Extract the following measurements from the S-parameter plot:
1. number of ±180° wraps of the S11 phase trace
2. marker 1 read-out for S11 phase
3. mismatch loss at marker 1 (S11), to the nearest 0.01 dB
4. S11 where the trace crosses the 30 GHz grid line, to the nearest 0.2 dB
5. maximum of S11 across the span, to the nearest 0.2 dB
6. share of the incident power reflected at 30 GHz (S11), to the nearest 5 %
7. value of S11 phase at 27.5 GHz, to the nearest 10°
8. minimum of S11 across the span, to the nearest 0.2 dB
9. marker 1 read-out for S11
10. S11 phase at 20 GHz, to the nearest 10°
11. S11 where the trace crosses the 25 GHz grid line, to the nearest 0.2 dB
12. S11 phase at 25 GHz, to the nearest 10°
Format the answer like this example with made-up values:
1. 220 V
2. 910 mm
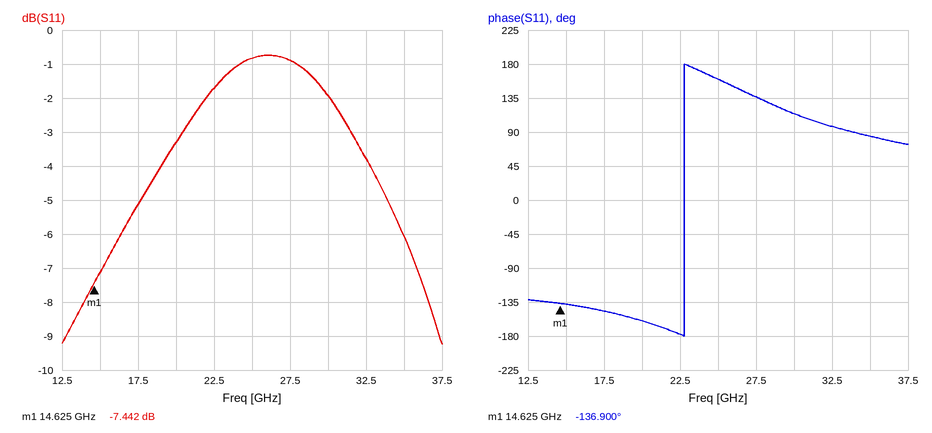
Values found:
1. 1
2. -136.900°
3. 0.86 dB
4. -2.0 dB
5. -0.8 dB
6. 65 %
7. 140°
8. -9.2 dB
9. -7.442 dB
10. -160°
11. -0.8 dB
12. 160°
